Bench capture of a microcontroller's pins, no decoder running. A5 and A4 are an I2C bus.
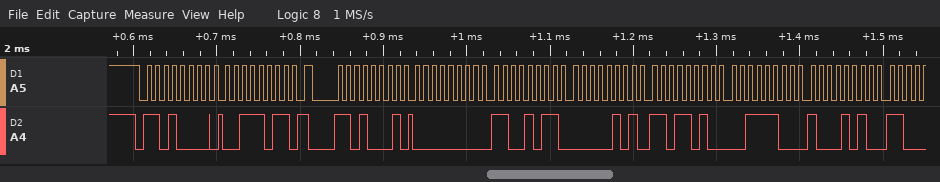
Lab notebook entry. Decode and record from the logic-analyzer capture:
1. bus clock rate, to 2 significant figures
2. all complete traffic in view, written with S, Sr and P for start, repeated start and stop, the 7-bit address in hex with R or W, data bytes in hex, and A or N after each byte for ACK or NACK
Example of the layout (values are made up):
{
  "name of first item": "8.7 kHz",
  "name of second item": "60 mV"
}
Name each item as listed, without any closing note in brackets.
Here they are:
{
  "bus clock rate, to 2 significant figures": "100 kHz",
  "all complete traffic in view, written with S, Sr and P for start, repeated start and stop, the 7-bit address in hex with R or W, data bytes in hex, and A or N after each byte for ACK or NACK": "S 68W A 3B A Sr 68R A 00 A CB A 05 A DA A 3C A 8A A"
}
